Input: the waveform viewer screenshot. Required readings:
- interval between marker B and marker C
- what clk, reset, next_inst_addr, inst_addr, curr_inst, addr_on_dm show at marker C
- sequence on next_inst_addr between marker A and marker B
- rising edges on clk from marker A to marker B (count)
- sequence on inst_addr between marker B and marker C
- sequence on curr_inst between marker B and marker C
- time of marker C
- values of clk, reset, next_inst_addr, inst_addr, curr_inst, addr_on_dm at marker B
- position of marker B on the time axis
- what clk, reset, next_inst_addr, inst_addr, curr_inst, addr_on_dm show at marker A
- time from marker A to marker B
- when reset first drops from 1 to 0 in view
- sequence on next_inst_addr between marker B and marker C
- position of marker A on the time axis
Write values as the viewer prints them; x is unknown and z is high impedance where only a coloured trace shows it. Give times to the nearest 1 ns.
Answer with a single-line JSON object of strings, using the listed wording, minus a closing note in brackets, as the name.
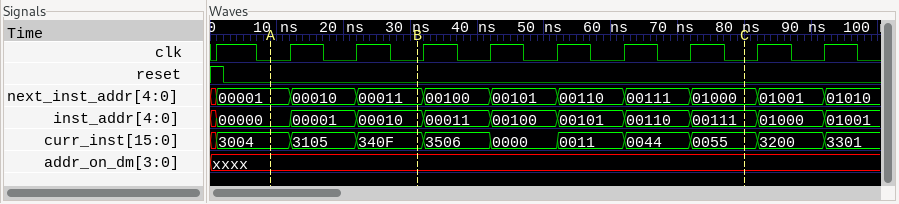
{"interval between marker B and marker C": "49 ns", "what clk, reset, next_inst_addr, inst_addr, curr_inst, addr_on_dm show at marker C": "clk=0, reset=0, next_inst_addr=01000, inst_addr=00111, curr_inst=0055, addr_on_dm=xxxx", "sequence on next_inst_addr between marker A and marker B": "00001, 00010, 00011", "rising edges on clk from marker A to marker B": "2", "sequence on inst_addr between marker B and marker C": "00010, 00011, 00100, 00101, 00110, 00111", "sequence on curr_inst between marker B and marker C": "340F, 3506, 0000, 0011, 0044, 0055", "time of marker C": "80 ns", "values of clk, reset, next_inst_addr, inst_addr, curr_inst, addr_on_dm at marker B": "clk=0, reset=0, next_inst_addr=00011, inst_addr=00010, curr_inst=340F, addr_on_dm=xxxx", "position of marker B on the time axis": "31 ns", "what clk, reset, next_inst_addr, inst_addr, curr_inst, addr_on_dm show at marker A": "clk=0, reset=0, next_inst_addr=00001, inst_addr=00000, curr_inst=3004, addr_on_dm=xxxx", "time from marker A to marker B": "22 ns", "when reset first drops from 1 to 0 in view": "2 ns", "sequence on next_inst_addr between marker B and marker C": "00011, 00100, 00101, 00110, 00111, 01000", "position of marker A on the time axis": "9 ns"}
